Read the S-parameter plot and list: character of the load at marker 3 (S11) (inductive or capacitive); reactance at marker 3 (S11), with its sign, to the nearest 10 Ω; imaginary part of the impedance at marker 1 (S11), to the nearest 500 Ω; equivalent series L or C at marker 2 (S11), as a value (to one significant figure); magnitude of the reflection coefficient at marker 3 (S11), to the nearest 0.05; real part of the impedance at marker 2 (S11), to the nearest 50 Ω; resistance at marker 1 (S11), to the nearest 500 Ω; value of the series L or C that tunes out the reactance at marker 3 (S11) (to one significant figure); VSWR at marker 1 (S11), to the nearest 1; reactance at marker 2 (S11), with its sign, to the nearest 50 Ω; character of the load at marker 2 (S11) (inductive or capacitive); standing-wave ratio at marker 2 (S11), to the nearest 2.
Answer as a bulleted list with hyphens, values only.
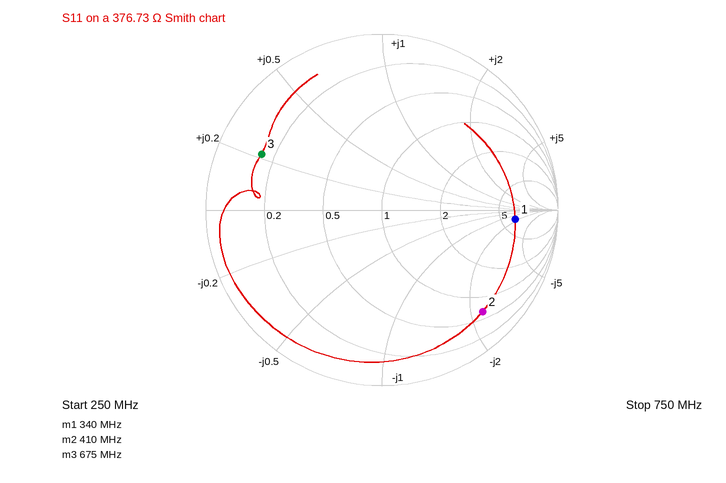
- inductive
- +80 Ω
- -500 Ω
- 500 fF
- 0.75
- 250 Ω
- 2500 Ω
- 3 pF
- 7
- -850 Ω
- capacitive
- 10
